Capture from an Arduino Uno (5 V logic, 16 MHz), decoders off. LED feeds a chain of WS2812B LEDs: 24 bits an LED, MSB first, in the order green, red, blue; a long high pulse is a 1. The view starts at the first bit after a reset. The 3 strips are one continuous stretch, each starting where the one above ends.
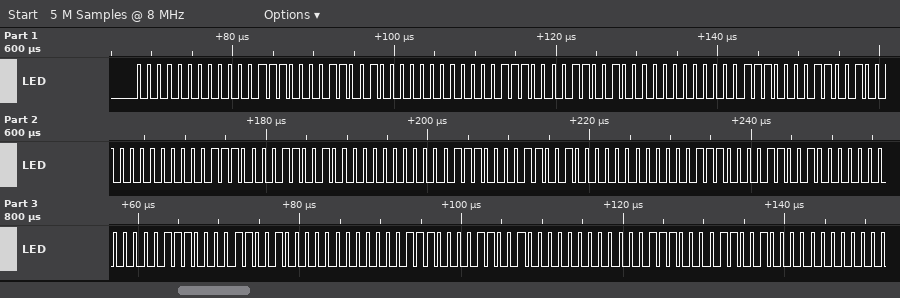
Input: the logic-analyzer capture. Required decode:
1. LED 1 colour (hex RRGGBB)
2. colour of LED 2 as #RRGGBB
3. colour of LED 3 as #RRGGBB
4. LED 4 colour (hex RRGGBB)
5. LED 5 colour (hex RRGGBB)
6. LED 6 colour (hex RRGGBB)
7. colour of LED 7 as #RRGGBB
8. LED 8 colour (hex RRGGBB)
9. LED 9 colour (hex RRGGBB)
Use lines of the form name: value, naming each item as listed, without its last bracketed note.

LED 1 colour: #0E0019
colour of LED 2 as #RRGGBB: #0E0019
colour of LED 3 as #RRGGBB: #0E0019
LED 4 colour: #0E0019
LED 5 colour: #0E0019
LED 6 colour: #0E0019
colour of LED 7 as #RRGGBB: #0E0019
LED 8 colour: #0E0019
LED 9 colour: #0E0019
